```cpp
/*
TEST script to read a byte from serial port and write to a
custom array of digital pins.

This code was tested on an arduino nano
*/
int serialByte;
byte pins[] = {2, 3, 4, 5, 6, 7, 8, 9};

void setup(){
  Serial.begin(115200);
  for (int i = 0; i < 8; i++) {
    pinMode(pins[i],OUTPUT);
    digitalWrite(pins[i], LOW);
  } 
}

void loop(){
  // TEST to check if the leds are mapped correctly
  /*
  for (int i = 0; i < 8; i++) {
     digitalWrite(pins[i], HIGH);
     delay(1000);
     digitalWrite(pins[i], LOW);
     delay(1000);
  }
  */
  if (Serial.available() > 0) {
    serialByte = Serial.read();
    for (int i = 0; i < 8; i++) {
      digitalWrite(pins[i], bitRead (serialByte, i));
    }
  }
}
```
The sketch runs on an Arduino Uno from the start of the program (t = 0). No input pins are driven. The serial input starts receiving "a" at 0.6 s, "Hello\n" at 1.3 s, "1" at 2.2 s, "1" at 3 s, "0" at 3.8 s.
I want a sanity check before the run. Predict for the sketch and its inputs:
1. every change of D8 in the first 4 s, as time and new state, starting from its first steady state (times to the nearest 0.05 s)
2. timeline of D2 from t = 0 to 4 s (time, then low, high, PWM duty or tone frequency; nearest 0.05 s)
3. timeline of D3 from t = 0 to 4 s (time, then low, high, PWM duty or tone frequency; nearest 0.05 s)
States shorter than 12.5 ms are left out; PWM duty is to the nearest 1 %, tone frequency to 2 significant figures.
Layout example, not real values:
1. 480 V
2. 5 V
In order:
1. 0 s low; 0.6 s high; 1.3 s low
2. 0 s low; 0.6 s high; 1.3 s low; 2.2 s high; 3.8 s low
3. 0 s low; 1.3 s high; 2.2 s low
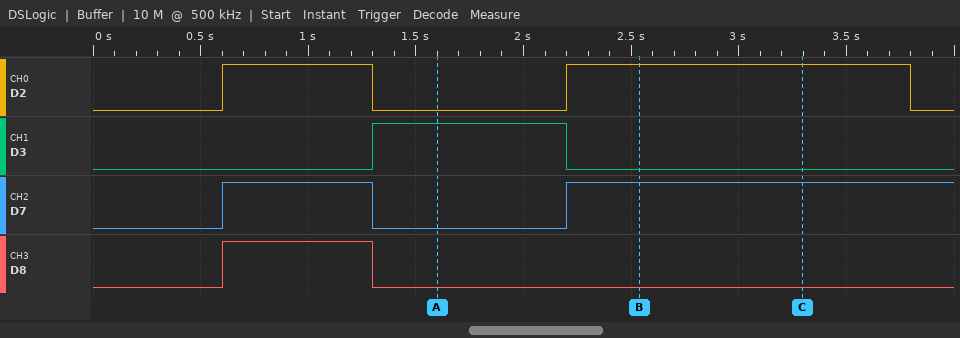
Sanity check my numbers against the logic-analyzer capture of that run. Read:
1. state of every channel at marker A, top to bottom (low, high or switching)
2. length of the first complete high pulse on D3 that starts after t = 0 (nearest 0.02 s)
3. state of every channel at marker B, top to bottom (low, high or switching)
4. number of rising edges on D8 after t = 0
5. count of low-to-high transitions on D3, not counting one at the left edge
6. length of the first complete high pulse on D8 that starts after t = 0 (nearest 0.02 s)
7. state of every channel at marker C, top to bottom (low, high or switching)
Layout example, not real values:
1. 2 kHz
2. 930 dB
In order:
1. D2 low, D3 high, D7 low, D8 low
2. 0.90 s
3. D2 high, D3 low, D7 high, D8 low
4. 1
5. 1
6. 0.70 s
7. D2 high, D3 low, D7 high, D8 low
